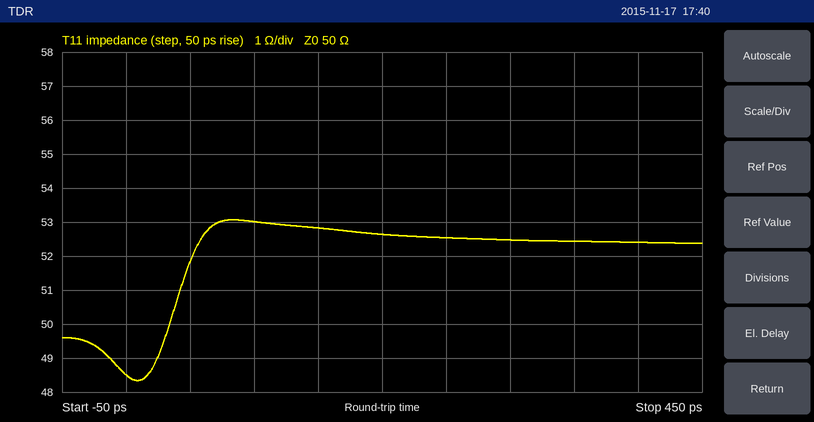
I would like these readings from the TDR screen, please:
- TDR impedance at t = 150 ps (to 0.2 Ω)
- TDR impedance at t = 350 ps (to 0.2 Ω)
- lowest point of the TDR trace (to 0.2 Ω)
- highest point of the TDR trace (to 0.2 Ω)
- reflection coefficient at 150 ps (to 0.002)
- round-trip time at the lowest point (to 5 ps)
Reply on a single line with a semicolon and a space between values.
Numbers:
52.8 Ω; 52.4 Ω; 48.4 Ω; 53.0 Ω; +0.028; 10 ps
